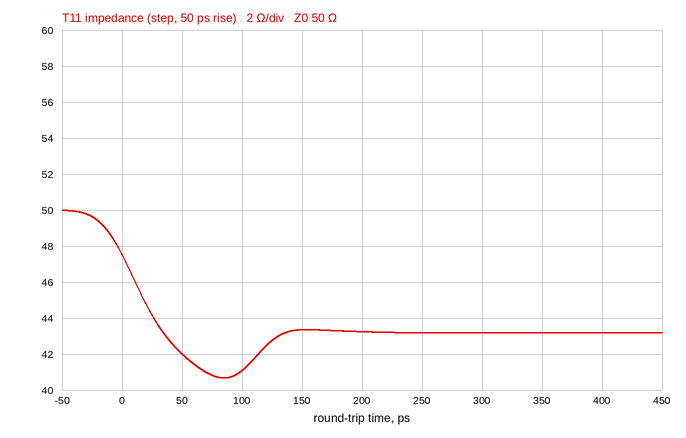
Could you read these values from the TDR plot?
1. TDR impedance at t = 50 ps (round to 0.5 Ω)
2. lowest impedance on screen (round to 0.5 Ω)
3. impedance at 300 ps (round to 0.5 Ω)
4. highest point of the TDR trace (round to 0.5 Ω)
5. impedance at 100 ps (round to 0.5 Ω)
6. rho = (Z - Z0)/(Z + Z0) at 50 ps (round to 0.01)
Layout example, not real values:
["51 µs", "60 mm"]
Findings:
["42.0 Ω", "40.5 Ω", "43.0 Ω", "50.0 Ω", "41.0 Ω", "-0.09"]
